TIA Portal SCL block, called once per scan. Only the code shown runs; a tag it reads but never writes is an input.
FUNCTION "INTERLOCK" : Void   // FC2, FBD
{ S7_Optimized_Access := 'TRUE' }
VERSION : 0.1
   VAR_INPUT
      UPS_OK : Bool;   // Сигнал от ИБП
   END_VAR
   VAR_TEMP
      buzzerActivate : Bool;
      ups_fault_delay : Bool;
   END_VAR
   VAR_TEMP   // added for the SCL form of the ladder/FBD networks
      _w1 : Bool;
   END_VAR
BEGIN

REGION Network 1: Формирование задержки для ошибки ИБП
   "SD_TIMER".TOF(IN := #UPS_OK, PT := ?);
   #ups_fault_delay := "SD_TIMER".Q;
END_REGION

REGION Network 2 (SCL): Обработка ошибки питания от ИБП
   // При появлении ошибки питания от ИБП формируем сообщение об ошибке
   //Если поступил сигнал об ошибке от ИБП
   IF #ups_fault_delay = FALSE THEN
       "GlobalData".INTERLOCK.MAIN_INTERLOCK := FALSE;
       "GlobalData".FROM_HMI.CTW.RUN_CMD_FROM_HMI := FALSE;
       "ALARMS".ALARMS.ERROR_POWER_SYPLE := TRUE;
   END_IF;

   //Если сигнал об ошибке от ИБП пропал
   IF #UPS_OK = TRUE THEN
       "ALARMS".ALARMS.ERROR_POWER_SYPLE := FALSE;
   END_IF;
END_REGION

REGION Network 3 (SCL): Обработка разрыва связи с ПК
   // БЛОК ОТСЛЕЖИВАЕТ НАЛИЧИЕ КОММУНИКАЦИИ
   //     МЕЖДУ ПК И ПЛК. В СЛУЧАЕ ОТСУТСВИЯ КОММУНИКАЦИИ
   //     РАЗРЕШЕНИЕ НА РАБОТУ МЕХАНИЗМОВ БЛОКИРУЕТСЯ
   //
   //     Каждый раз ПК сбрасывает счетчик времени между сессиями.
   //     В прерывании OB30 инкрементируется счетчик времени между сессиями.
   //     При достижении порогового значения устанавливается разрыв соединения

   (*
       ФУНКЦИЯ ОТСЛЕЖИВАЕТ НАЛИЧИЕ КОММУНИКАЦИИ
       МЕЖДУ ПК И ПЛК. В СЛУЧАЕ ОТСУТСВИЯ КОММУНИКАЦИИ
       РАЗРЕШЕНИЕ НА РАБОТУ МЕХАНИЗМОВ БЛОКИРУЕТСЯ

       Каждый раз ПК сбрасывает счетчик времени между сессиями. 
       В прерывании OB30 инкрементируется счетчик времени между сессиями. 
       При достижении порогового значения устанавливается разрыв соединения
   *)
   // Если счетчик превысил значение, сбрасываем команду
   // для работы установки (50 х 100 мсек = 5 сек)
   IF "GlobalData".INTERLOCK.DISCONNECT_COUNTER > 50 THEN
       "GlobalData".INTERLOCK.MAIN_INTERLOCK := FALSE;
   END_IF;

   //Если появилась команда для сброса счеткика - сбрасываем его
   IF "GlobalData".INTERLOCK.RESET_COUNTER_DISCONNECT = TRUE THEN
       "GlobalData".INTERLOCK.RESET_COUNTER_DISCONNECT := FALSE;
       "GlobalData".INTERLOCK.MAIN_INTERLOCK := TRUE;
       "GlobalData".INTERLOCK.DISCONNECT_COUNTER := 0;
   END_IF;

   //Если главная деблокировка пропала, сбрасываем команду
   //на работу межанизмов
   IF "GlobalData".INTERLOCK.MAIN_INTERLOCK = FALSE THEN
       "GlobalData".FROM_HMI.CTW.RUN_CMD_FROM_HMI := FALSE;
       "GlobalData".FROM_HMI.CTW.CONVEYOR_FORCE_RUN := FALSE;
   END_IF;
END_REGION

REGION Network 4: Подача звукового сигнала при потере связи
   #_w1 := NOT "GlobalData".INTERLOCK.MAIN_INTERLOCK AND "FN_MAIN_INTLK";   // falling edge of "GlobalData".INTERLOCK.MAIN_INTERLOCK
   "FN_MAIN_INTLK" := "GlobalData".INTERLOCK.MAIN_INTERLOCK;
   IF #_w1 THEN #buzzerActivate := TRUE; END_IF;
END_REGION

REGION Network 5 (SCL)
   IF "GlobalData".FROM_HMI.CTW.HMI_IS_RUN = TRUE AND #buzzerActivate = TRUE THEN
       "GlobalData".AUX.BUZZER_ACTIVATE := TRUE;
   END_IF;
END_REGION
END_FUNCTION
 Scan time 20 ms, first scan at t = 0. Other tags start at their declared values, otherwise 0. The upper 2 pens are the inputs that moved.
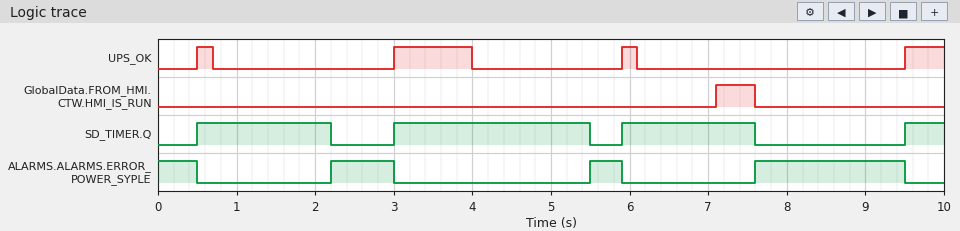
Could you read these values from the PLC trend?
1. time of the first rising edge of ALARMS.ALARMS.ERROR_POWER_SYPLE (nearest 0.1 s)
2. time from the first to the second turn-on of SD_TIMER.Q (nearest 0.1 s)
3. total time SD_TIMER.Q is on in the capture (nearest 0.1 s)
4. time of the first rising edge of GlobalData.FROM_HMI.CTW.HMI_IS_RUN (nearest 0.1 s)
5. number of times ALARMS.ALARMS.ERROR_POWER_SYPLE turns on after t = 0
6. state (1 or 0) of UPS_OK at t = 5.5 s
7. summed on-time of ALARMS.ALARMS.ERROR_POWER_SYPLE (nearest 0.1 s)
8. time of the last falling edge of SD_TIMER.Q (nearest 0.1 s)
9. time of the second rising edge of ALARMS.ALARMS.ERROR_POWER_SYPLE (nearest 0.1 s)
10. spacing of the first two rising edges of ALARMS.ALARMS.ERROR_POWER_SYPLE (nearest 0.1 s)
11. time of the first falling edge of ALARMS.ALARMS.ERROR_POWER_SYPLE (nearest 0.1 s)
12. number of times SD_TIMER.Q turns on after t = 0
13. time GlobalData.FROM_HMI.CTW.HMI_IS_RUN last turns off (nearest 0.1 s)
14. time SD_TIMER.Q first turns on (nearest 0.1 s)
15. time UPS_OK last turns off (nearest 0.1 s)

2.2 s
2.5 s
6.4 s
7.1 s
3
0
3.6 s
7.6 s
5.5 s
3.3 s
0.5 s
4
7.6 s
0.5 s
6.1 s
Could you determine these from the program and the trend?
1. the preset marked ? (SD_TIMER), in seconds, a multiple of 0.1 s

1.5 s
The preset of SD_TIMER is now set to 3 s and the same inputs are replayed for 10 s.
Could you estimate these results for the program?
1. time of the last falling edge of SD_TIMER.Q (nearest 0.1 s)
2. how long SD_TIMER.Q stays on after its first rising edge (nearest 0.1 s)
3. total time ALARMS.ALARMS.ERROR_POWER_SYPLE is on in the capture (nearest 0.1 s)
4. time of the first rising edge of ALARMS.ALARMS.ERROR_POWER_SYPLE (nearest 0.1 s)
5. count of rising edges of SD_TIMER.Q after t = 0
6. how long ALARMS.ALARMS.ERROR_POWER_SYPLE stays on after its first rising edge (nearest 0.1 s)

9.1 s
8.6 s
0.9 s
9.1 s
2
0.4 s
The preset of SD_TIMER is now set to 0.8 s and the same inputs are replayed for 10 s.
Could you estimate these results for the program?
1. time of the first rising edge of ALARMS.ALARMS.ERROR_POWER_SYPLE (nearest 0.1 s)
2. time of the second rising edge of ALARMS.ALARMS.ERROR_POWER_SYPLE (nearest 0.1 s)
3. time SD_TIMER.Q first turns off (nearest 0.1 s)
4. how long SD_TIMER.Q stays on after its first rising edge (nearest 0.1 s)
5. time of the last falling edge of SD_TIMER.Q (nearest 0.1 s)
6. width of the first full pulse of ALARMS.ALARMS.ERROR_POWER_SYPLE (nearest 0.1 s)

1.5 s
4.8 s
1.5 s
1.0 s
6.9 s
1.5 s
